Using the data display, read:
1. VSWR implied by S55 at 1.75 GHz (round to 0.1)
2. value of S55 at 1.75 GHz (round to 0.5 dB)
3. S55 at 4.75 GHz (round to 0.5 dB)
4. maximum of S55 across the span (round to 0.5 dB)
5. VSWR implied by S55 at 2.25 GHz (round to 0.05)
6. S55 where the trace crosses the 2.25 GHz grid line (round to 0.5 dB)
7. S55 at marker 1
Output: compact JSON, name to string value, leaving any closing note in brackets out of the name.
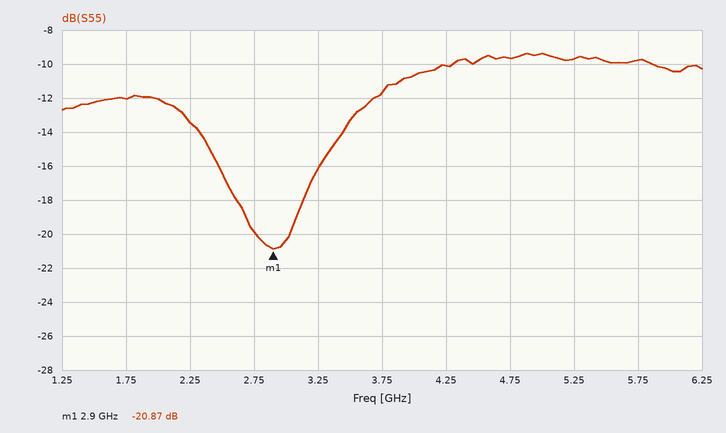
{"VSWR implied by S55 at 1.75 GHz": "1.7", "value of S55 at 1.75 GHz": "-12.0 dB", "S55 at 4.75 GHz": "-9.5 dB", "maximum of S55 across the span": "-9.5 dB", "VSWR implied by S55 at 2.25 GHz": "1.55", "S55 where the trace crosses the 2.25 GHz grid line": "-13.5 dB", "S55 at marker 1": "-20.87 dB"}
